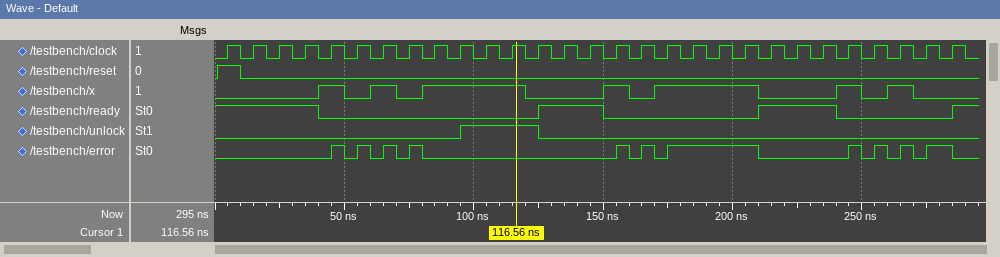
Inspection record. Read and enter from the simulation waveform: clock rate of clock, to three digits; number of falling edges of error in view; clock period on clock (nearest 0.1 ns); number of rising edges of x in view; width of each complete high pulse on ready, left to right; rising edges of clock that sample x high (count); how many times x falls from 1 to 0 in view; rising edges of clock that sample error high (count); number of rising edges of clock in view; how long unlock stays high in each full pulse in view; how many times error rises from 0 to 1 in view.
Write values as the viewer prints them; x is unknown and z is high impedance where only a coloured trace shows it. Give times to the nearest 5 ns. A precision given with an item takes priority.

100 MHz
11
10 ns
7
25 ns, 30 ns
13
7
4
29
30 ns
11
